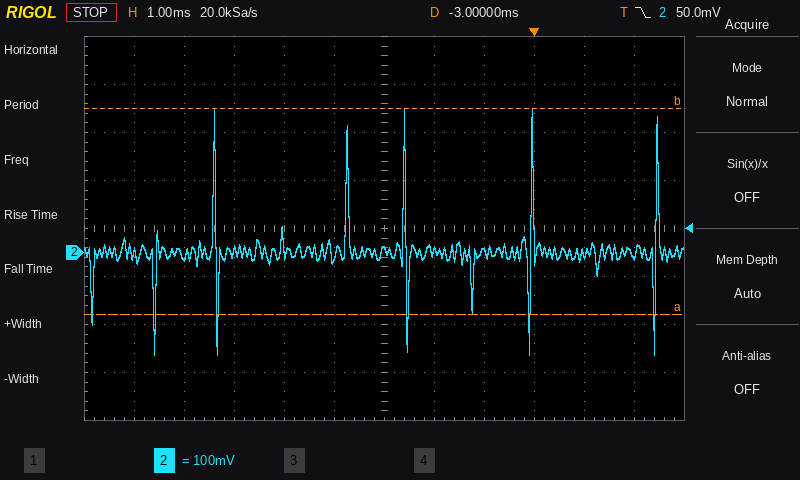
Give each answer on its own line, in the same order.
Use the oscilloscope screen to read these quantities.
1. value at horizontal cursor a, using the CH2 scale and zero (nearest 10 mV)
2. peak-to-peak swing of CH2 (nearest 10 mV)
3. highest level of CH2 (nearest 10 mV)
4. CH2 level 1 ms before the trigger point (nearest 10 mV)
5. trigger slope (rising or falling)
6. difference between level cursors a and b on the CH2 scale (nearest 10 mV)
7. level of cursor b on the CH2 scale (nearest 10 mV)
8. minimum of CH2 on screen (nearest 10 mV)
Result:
-130 mV
510 mV
300 mV
0 mV
falling
430 mV
300 mV
-210 mV
